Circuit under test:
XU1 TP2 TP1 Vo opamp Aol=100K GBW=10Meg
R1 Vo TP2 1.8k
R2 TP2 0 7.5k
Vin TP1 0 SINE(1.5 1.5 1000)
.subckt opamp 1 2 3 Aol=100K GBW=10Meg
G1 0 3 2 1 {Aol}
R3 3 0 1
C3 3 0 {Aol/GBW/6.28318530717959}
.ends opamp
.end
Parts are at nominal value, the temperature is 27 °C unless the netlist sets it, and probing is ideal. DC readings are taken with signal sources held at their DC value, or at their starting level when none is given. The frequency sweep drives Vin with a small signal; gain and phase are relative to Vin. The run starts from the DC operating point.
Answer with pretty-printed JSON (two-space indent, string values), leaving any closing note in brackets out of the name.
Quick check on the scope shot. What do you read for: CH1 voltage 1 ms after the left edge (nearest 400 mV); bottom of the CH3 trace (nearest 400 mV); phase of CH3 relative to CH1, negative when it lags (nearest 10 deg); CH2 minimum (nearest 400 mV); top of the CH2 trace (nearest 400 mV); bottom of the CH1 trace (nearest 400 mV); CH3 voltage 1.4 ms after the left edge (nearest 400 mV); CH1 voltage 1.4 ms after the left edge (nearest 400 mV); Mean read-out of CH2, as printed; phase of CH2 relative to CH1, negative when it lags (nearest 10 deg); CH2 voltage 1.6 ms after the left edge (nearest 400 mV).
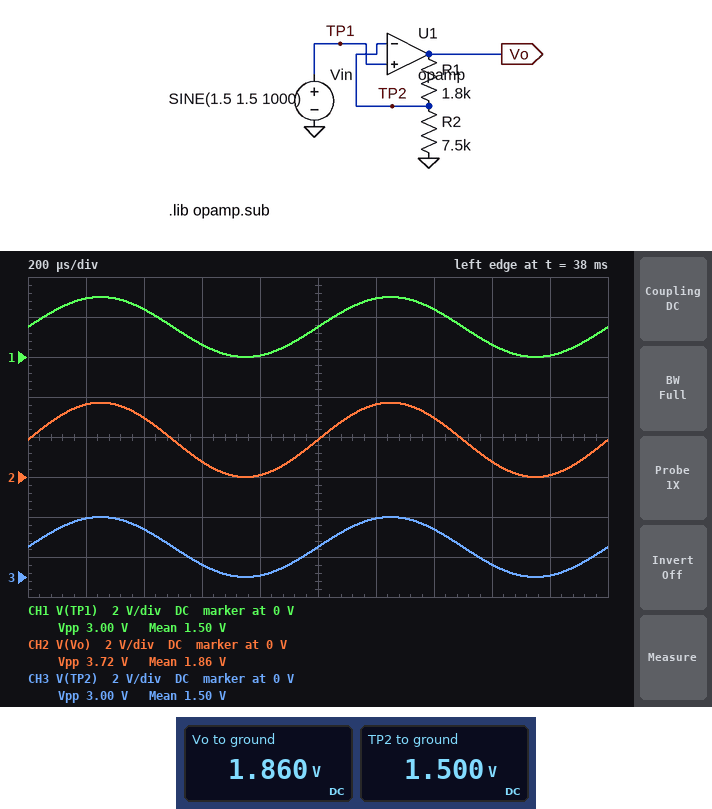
{
  "CH1 voltage 1 ms after the left edge": "1.6 V",
  "bottom of the CH3 trace": "0 V",
  "phase of CH3 relative to CH1, negative when it lags": "0 deg",
  "CH2 minimum": "0 V",
  "top of the CH2 trace": "3.6 V",
  "bottom of the CH1 trace": "0 V",
  "CH3 voltage 1.4 ms after the left edge": "2.4 V",
  "CH1 voltage 1.4 ms after the left edge": "2.4 V",
  "Mean read-out of CH2, as printed": "1.86 V",
  "phase of CH2 relative to CH1, negative when it lags": "0 deg",
  "CH2 voltage 1.6 ms after the left edge": "800 mV"
}
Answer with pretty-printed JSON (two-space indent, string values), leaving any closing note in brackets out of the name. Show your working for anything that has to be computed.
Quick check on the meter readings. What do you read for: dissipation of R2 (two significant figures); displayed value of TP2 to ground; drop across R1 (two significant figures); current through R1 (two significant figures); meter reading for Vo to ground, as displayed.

{
  "dissipation of R2": "(1.5 V)^2 / 7.5 kΩ = 300 µW",
  "displayed value of TP2 to ground": "1.500 V",
  "drop across R1": "1.86 V - 1.5 V = 360 mV",
  "current through R1": "(1.86 V - 1.5 V) / 1.8 kΩ = 200 µA",
  "meter reading for Vo to ground, as displayed": "1.860 V"
}
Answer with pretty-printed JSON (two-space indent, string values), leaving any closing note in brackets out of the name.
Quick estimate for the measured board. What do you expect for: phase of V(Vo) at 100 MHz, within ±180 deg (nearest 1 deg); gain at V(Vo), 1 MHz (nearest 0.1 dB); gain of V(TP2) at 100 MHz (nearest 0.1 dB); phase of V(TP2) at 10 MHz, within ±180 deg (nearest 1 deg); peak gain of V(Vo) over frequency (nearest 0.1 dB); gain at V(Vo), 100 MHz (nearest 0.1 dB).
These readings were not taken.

{
  "phase of V(Vo) at 100 MHz, within ±180 deg": "-85 deg",
  "gain at V(Vo), 1 MHz": "1.8 dB",
  "gain of V(TP2) at 100 MHz": "-21.9 dB",
  "phase of V(TP2) at 10 MHz, within ±180 deg": "-51 deg",
  "peak gain of V(Vo) over frequency": "1.9 dB",
  "gain at V(Vo), 100 MHz": "-20.0 dB"
}
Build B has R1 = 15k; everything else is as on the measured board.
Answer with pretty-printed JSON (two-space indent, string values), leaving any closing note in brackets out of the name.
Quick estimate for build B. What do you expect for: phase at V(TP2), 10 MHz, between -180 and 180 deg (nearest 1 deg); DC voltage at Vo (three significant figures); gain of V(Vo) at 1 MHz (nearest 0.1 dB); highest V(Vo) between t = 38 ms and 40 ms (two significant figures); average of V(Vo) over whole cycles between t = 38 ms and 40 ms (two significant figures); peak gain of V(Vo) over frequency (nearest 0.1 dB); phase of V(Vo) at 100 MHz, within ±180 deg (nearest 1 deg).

{
  "phase at V(TP2), 10 MHz, between -180 and 180 deg": "-72 deg",
  "DC voltage at Vo": "4.50 V",
  "gain of V(Vo) at 1 MHz": "9.2 dB",
  "highest V(Vo) between t = 38 ms and 40 ms": "9.0 V",
  "average of V(Vo) over whole cycles between t = 38 ms and 40 ms": "4.5 V",
  "peak gain of V(Vo) over frequency": "9.5 dB",
  "phase of V(Vo) at 100 MHz, within ±180 deg": "-88 deg"
}
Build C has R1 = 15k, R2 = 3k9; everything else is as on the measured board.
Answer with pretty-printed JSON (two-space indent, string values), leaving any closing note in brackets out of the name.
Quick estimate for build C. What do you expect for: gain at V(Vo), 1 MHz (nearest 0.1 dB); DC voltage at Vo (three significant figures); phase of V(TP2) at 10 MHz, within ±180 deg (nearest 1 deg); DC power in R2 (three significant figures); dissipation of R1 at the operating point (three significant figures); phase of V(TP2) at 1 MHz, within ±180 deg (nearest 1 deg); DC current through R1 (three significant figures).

{
  "gain at V(Vo), 1 MHz": "12.8 dB",
  "DC voltage at Vo": "7.27 V",
  "phase of V(TP2) at 10 MHz, within ±180 deg": "-78 deg",
  "DC power in R2": "577 µW",
  "dissipation of R1 at the operating point": "2.22 mW",
  "phase of V(TP2) at 1 MHz, within ±180 deg": "-26 deg",
  "DC current through R1": "385 µA"
}
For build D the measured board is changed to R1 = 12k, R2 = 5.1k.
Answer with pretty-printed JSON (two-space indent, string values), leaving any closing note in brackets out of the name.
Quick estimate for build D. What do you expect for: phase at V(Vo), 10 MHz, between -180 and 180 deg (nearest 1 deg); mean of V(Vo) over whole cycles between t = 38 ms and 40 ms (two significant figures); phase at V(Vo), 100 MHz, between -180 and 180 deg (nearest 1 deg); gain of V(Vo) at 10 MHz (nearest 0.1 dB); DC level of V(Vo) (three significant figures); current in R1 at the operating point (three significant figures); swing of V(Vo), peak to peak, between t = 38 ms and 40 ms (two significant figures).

{
  "phase at V(Vo), 10 MHz, between -180 and 180 deg": "-73 deg",
  "mean of V(Vo) over whole cycles between t = 38 ms and 40 ms": "5.0 V",
  "phase at V(Vo), 100 MHz, between -180 and 180 deg": "-88 deg",
  "gain of V(Vo) at 10 MHz": "-0.4 dB",
  "DC level of V(Vo)": "5.03 V",
  "current in R1 at the operating point": "294 µA",
  "swing of V(Vo), peak to peak, between t = 38 ms and 40 ms": "10 V"
}
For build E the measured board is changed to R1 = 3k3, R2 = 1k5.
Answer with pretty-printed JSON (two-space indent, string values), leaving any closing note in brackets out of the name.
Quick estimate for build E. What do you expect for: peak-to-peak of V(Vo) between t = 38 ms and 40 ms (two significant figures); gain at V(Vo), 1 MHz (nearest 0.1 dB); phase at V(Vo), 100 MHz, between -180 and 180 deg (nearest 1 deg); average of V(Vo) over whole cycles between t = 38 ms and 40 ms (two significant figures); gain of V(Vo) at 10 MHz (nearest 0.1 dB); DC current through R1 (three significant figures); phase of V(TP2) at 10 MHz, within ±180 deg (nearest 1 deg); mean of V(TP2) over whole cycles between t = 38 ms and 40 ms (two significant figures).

{
  "peak-to-peak of V(Vo) between t = 38 ms and 40 ms": "9.6 V",
  "gain at V(Vo), 1 MHz": "9.7 dB",
  "phase at V(Vo), 100 MHz, between -180 and 180 deg": "-88 deg",
  "average of V(Vo) over whole cycles between t = 38 ms and 40 ms": "4.8 V",
  "gain of V(Vo) at 10 MHz": "-0.4 dB",
  "DC current through R1": "1.00 mA",
  "phase of V(TP2) at 10 MHz, within ±180 deg": "-73 deg",
  "mean of V(TP2) over whole cycles between t = 38 ms and 40 ms": "1.5 V"
}
